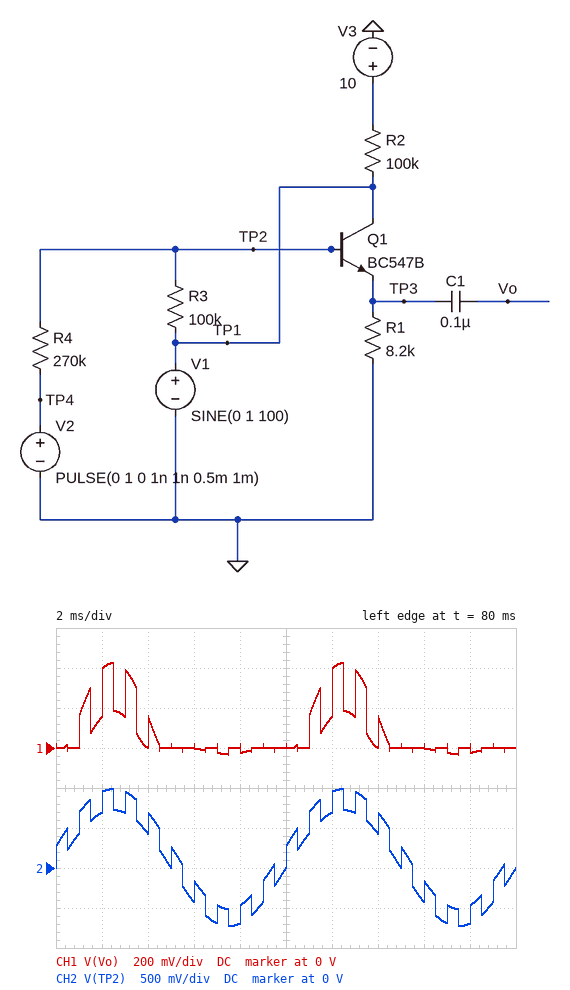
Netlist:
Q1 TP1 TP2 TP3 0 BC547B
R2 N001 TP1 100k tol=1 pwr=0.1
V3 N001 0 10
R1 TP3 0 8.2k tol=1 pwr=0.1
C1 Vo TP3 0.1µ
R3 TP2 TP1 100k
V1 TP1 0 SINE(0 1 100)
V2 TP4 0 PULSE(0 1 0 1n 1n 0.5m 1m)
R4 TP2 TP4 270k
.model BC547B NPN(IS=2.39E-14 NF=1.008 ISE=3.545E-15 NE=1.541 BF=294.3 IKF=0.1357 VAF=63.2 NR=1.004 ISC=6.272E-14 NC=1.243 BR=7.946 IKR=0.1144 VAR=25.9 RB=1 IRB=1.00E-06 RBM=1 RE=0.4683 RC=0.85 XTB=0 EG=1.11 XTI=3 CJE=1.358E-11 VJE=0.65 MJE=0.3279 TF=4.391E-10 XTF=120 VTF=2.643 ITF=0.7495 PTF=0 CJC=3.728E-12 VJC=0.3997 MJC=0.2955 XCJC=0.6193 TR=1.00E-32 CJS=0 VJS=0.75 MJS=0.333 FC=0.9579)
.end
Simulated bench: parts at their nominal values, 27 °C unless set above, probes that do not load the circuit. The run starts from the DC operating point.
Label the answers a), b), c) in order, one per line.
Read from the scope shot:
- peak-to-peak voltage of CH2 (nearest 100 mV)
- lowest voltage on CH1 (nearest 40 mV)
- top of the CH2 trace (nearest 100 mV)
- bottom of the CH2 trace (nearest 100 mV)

a) 1.7 V
b) -40 mV
c) 1.0 V
d) -700 mV
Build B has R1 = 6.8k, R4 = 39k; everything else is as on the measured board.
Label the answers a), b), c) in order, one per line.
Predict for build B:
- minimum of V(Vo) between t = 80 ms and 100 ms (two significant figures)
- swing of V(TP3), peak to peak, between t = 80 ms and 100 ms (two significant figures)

a) -960 mV
b) 1.4 V
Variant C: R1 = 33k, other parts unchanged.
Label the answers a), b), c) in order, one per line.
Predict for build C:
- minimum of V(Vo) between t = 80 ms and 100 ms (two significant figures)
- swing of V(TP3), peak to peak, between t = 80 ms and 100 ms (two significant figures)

a) -120 mV
b) 590 mV
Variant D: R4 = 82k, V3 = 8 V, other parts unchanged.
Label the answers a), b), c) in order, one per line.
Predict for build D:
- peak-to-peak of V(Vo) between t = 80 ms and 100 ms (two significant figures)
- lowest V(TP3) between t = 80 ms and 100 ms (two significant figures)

a) 1.0 V
b) -580 mV
